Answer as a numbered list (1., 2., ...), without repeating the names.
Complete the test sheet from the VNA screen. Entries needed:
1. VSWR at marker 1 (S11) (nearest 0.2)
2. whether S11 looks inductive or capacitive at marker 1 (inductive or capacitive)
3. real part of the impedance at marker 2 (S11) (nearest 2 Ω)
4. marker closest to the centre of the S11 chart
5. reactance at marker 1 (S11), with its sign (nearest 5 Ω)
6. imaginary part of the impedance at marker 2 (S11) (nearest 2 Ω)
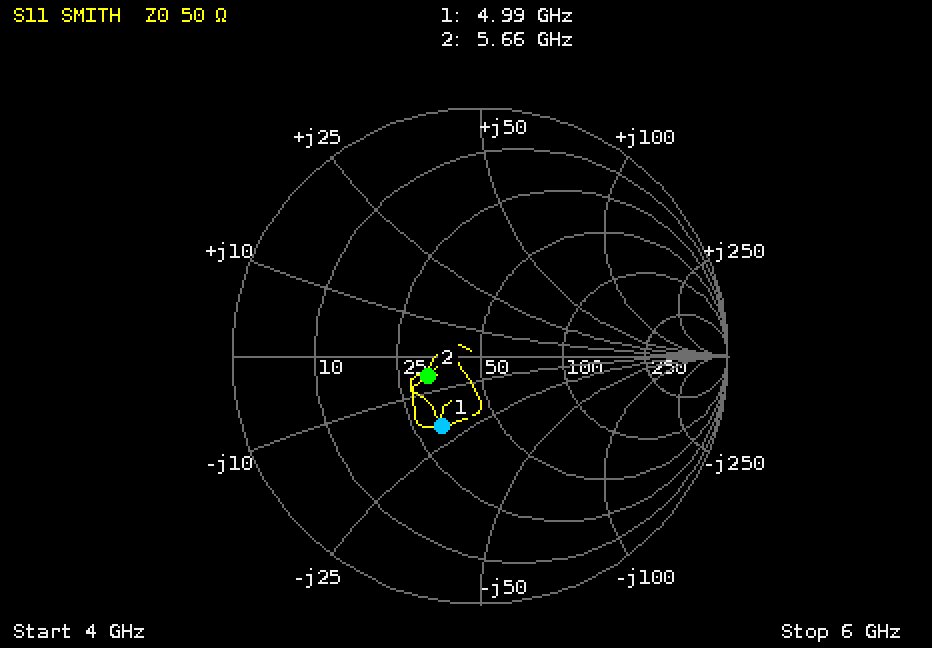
1. 2.0
2. capacitive
3. 32 Ω
4. marker 2
5. -20 Ω
6. -6 Ω
